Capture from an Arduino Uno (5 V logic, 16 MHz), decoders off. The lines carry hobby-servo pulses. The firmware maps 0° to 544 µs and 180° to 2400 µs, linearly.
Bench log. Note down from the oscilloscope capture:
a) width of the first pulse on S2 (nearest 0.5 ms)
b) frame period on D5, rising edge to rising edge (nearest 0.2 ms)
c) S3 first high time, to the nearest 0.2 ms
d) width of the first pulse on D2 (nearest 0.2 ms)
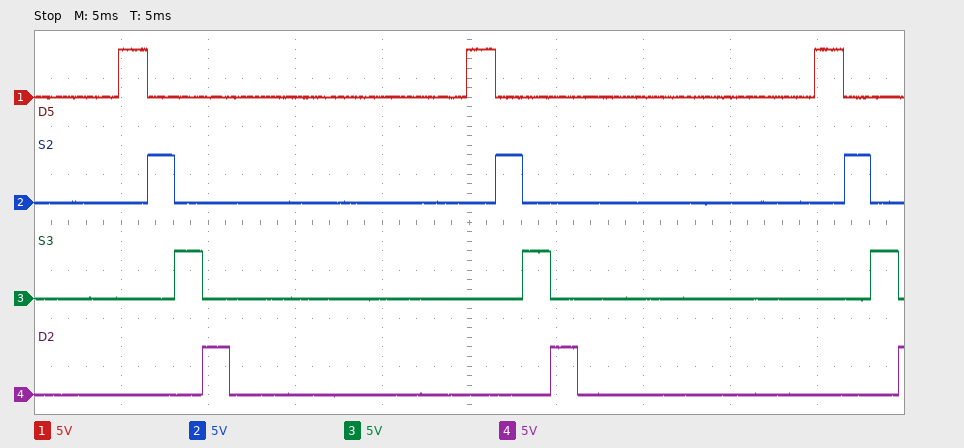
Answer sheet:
1.5 ms
20.0 ms
1.6 ms
1.6 ms
